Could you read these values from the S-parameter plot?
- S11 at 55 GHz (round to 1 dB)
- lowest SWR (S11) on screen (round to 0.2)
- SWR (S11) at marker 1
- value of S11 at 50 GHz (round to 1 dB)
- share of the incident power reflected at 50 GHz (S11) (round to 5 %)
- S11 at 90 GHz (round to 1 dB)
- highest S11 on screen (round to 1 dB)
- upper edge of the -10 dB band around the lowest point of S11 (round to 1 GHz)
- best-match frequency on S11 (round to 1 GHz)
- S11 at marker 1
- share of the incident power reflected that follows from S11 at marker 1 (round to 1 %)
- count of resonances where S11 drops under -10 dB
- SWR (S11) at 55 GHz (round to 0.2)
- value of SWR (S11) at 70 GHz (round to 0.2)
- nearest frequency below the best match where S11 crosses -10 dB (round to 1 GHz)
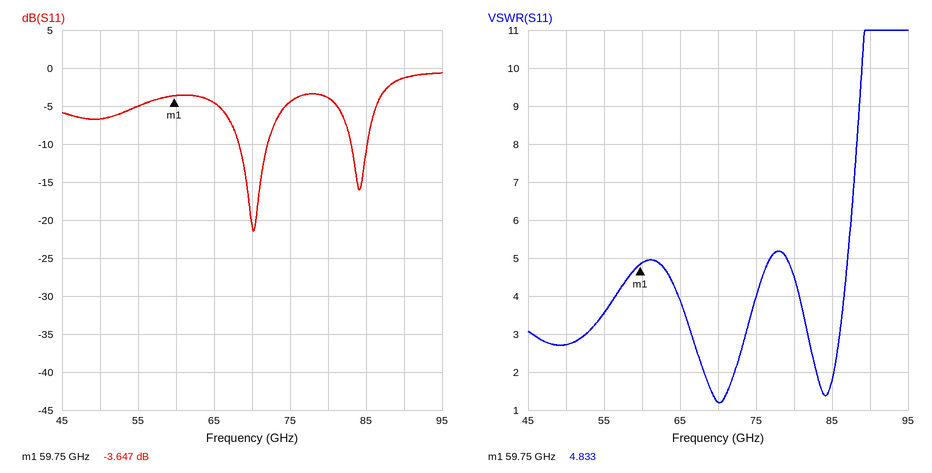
-5 dB
1.2
4.833
-7 dB
20 %
-1 dB
-1 dB
72 GHz
70 GHz
-3.647 dB
43 %
2
3.6
1.2
68 GHz
